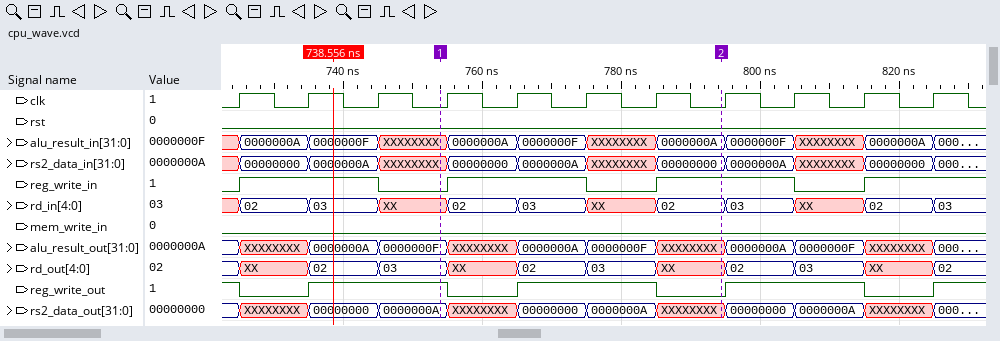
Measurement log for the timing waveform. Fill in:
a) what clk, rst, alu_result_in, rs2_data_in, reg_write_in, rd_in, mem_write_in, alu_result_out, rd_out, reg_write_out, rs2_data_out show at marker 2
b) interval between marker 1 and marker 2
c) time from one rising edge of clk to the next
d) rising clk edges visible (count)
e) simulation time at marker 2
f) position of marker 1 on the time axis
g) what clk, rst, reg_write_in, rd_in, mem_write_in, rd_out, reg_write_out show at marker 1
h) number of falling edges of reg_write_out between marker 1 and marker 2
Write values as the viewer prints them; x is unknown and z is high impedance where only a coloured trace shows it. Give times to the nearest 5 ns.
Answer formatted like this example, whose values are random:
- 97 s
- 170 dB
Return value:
- clk=0, rst=0, alu_result_in=0000000A, rs2_data_in=00000000, reg_write_in=1, rd_in=02, mem_write_in=0, alu_result_out=XXXXXXXX, rd_out=XX, reg_write_out=0, rs2_data_out=XXXXXXXX
- 40 ns
- 10 ns
- 11
- 795 ns
- 755 ns
- clk=0, rst=0, reg_write_in=0, rd_in=XX, mem_write_in=0, rd_out=03, reg_write_out=1
- 2
